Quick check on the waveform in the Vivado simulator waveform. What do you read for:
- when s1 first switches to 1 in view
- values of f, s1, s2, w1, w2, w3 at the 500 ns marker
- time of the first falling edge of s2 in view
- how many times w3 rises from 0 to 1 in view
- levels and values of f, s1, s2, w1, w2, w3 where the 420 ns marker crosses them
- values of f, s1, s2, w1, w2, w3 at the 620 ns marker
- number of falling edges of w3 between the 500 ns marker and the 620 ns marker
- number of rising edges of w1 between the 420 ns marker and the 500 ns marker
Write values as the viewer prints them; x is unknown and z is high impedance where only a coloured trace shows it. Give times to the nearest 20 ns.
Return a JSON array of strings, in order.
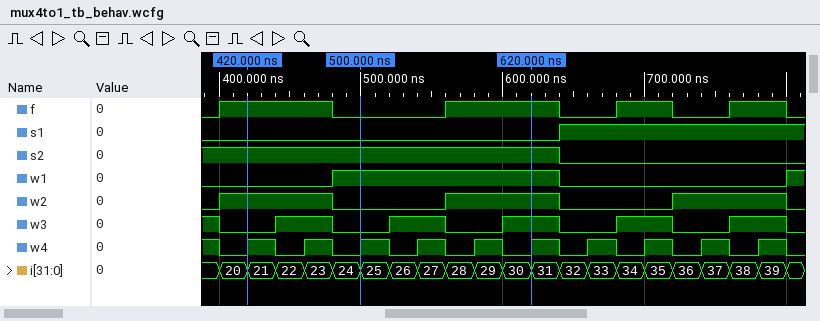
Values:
["640 ns", "f=0, s1=0, s2=1, w1=1, w2=0, w3=0", "640 ns", "5", "f=1, s1=0, s2=1, w1=0, w2=1, w3=0", "f=1, s1=0, s2=1, w1=1, w2=1, w3=1", "1", "1"]
